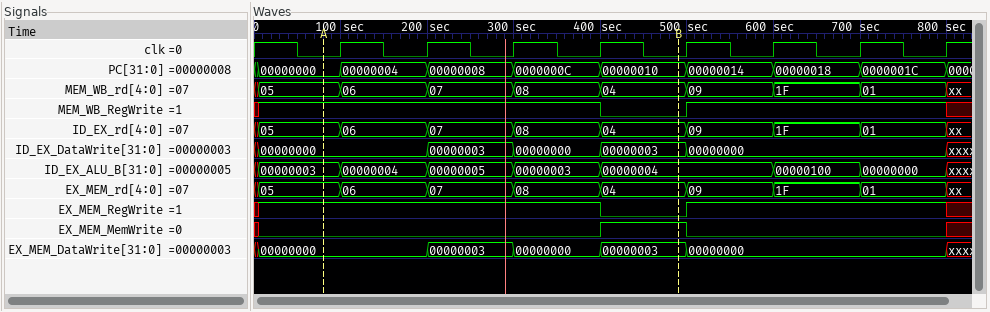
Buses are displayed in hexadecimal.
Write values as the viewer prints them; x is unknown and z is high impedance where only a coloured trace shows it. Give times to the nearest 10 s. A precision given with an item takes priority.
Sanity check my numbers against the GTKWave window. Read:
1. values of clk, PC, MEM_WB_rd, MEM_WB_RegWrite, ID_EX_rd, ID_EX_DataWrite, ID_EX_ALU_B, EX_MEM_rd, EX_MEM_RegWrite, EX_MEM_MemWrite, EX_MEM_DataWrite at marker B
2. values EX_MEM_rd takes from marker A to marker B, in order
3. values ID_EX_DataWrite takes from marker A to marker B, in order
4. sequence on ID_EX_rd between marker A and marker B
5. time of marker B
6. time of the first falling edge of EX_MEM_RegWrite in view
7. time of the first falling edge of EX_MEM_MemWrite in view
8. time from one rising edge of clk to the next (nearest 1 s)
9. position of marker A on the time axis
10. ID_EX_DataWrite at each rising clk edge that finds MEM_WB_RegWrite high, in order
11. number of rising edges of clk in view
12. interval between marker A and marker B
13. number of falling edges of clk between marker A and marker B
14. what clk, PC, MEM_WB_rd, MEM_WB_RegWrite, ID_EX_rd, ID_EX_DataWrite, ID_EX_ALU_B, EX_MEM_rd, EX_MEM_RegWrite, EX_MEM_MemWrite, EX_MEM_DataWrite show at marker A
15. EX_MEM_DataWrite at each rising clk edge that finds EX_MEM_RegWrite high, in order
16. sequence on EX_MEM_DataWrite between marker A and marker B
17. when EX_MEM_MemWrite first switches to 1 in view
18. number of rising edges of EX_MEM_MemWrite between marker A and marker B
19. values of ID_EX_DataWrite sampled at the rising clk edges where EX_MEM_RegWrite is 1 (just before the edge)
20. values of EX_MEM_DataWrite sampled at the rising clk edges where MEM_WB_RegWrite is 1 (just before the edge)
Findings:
clk=0, PC=00000010, MEM_WB_rd=04, MEM_WB_RegWrite=0, ID_EX_rd=04, ID_EX_DataWrite=00000003, ID_EX_ALU_B=00000004, EX_MEM_rd=04, EX_MEM_RegWrite=0, EX_MEM_MemWrite=1, EX_MEM_DataWrite=00000003
05, 06, 07, 08, 04
00000000, 00000003, 00000000, 00000003
05, 06, 07, 08, 04
490 s
400 s
500 s
100 s
80 s
00000000, 00000000, 00000003, 00000000, 00000000, 00000000, 00000000
8
410 s
4
clk=0, PC=00000000, MEM_WB_rd=05, MEM_WB_RegWrite=1, ID_EX_rd=05, ID_EX_DataWrite=00000000, ID_EX_ALU_B=00000003, EX_MEM_rd=05, EX_MEM_RegWrite=1, EX_MEM_MemWrite=0, EX_MEM_DataWrite=00000000
00000000, 00000000, 00000003, 00000000, 00000000, 00000000, 00000000
00000000, 00000003, 00000000, 00000003
400 s
1
00000000, 00000000, 00000003, 00000000, 00000000, 00000000, 00000000
00000000, 00000000, 00000003, 00000000, 00000000, 00000000, 00000000
